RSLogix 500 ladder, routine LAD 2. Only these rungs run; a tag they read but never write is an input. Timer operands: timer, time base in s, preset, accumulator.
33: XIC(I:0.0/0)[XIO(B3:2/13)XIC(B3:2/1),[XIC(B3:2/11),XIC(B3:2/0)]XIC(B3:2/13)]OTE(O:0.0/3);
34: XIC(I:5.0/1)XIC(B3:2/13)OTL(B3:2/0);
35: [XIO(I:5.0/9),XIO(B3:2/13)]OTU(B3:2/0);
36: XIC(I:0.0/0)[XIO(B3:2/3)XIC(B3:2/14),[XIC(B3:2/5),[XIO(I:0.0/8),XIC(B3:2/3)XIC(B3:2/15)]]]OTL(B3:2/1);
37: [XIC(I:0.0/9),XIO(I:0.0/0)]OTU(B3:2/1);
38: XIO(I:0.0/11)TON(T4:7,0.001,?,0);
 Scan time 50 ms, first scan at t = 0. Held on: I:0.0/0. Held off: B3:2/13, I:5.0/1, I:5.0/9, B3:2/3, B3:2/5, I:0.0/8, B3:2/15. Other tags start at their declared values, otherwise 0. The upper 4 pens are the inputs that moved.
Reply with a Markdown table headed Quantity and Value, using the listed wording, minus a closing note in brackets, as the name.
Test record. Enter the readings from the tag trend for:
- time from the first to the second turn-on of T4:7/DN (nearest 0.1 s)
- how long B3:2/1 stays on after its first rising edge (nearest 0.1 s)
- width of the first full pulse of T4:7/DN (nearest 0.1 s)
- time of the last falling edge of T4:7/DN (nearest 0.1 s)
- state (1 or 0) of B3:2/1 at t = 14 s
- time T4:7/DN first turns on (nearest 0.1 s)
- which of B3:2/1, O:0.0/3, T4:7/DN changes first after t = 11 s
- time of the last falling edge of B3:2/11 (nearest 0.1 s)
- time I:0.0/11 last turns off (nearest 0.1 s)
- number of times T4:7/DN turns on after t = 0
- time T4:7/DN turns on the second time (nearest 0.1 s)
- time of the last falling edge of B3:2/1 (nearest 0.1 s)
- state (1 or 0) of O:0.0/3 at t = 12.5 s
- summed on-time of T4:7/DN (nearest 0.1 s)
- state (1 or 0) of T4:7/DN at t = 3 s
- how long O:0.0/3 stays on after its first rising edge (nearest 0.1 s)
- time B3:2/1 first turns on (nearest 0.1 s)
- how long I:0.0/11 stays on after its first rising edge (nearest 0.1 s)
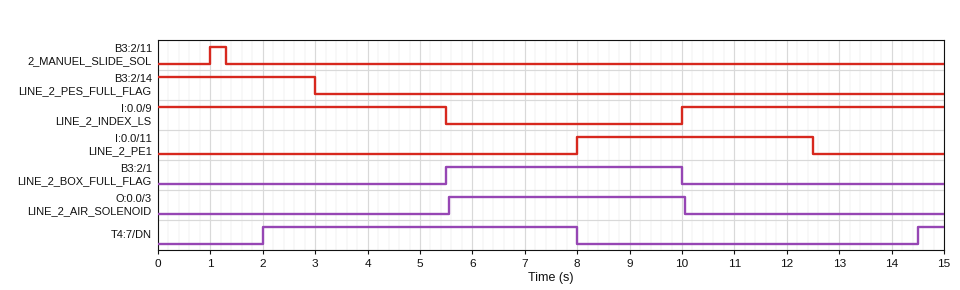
| Quantity | Value |
|---|---|
| time from the first to the second turn-on of T4:7/DN | 12.5 s |
| how long B3:2/1 stays on after its first rising edge | 4.5 s |
| width of the first full pulse of T4:7/DN | 6.0 s |
| time of the last falling edge of T4:7/DN | 8.0 s |
| state (1 or 0) of B3:2/1 at t = 14 s | 0 |
| time T4:7/DN first turns on | 2.0 s |
| which of B3:2/1, O:0.0/3, T4:7/DN changes first after t = 11 s | T4:7/DN |
| time of the last falling edge of B3:2/11 | 1.3 s |
| time I:0.0/11 last turns off | 12.5 s |
| number of times T4:7/DN turns on after t = 0 | 2 |
| time T4:7/DN turns on the second time | 14.5 s |
| time of the last falling edge of B3:2/1 | 10.0 s |
| state (1 or 0) of O:0.0/3 at t = 12.5 s | 0 |
| summed on-time of T4:7/DN | 6.5 s |
| state (1 or 0) of T4:7/DN at t = 3 s | 1 |
| how long O:0.0/3 stays on after its first rising edge | 4.5 s |
| time B3:2/1 first turns on | 5.5 s |
| how long I:0.0/11 stays on after its first rising edge | 4.5 s |
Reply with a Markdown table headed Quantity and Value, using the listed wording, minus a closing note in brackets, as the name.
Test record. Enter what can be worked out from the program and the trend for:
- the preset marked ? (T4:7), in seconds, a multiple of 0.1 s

| Quantity | Value |
|---|---|
| the preset marked ? (T4:7), in seconds, a multiple of 0.1 s | 2.0 s |
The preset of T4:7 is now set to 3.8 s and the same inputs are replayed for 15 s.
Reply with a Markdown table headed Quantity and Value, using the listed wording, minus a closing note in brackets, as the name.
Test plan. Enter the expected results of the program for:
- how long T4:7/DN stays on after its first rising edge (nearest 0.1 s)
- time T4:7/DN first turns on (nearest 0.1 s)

| Quantity | Value |
|---|---|
| how long T4:7/DN stays on after its first rising edge | 4.2 s |
| time T4:7/DN first turns on | 3.8 s |
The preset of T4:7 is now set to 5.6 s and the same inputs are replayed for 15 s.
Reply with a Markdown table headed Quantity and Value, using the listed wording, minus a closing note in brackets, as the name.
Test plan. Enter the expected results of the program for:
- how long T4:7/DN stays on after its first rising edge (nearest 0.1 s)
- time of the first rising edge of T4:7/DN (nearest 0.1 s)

| Quantity | Value |
|---|---|
| how long T4:7/DN stays on after its first rising edge | 2.4 s |
| time of the first rising edge of T4:7/DN | 5.6 s |
